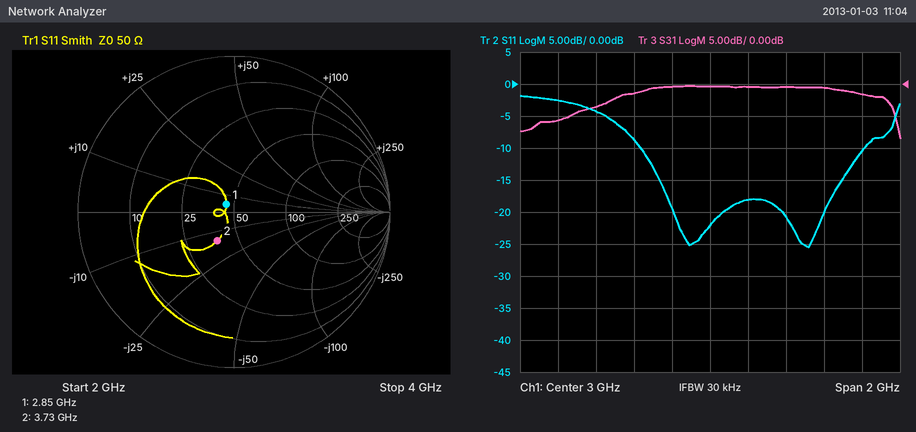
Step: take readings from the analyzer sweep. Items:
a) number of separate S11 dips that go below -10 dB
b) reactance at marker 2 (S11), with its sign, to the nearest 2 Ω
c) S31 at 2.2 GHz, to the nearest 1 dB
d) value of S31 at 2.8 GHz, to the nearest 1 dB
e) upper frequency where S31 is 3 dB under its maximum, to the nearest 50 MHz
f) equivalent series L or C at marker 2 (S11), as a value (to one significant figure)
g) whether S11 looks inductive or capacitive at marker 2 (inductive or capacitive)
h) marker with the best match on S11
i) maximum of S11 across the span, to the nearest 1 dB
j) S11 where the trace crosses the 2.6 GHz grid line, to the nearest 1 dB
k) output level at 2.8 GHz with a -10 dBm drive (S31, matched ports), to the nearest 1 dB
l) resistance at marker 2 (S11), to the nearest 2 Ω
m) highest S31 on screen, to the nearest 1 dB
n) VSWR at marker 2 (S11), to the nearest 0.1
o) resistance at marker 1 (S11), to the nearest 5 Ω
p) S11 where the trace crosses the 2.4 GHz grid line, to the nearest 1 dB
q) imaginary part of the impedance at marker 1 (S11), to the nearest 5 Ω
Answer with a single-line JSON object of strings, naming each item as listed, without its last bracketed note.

{"number of separate S11 dips that go below -10 dB": "2", "reactance at marker 2 (S11), with its sign, to the nearest 2 Ω": "-14 Ω", "S31 at 2.2 GHz, to the nearest 1 dB": "-6 dB", "value of S31 at 2.8 GHz, to the nearest 1 dB": "0 dB", "upper frequency where S31 is 3 dB under its maximum, to the nearest 50 MHz": "3.95 GHz", "equivalent series L or C at marker 2 (S11), as a value": "3 pF", "whether S11 looks inductive or capacitive at marker 2": "capacitive", "marker with the best match on S11": "marker 1", "maximum of S11 across the span, to the nearest 1 dB": "-2 dB", "S11 where the trace crosses the 2.6 GHz grid line, to the nearest 1 dB": "-9 dB", "output level at 2.8 GHz with a -10 dBm drive (S31, matched ports), to the nearest 1 dB": "-10 dBm", "resistance at marker 2 (S11), to the nearest 2 Ω": "38 Ω", "highest S31 on screen, to the nearest 1 dB": "0 dB", "VSWR at marker 2 (S11), to the nearest 0.1": "1.5", "resistance at marker 1 (S11), to the nearest 5 Ω": "45 Ω", "S11 where the trace crosses the 2.4 GHz grid line, to the nearest 1 dB": "-4 dB", "imaginary part of the impedance at marker 1 (S11), to the nearest 5 Ω": "+5 Ω"}
